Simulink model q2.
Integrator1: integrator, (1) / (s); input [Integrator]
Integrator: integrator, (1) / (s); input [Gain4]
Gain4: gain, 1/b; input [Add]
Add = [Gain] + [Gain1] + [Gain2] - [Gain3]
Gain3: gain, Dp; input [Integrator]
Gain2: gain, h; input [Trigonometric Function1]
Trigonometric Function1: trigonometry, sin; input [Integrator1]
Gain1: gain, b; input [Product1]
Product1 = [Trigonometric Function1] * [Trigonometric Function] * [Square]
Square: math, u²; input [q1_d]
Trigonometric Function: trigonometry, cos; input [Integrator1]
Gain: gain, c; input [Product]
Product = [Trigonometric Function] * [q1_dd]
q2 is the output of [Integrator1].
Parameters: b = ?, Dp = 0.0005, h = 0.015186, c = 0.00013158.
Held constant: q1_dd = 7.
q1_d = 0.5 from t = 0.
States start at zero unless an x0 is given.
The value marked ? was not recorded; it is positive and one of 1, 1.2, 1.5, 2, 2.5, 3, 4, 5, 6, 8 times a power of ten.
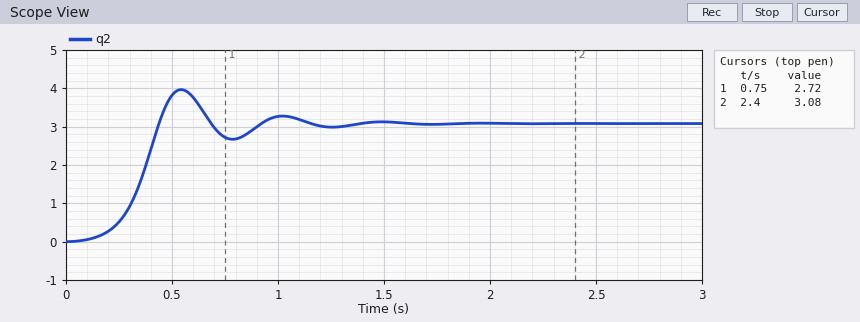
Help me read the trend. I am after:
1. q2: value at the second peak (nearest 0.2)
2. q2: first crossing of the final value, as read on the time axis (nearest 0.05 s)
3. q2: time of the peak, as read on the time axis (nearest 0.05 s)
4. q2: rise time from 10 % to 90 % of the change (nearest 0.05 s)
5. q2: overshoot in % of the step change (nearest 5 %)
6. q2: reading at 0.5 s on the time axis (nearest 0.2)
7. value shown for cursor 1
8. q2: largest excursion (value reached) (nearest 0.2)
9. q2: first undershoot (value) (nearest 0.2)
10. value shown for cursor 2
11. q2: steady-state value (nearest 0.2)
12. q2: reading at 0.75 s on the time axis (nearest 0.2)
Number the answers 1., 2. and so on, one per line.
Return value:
1. 3.2
2. 0.45 s
3. 0.55 s
4. 0.20 s
5. 30 %
6. 3.8
7. 2.72
8. 4.0
9. 2.6
10. 3.08
11. 3.0
12. 2.8
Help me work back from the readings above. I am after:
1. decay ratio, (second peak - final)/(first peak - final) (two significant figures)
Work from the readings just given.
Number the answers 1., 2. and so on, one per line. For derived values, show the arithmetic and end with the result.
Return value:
1. (3.2 - 3) / (4 - 3) = 0.20
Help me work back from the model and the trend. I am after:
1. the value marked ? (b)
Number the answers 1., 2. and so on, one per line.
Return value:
1. 8e-05
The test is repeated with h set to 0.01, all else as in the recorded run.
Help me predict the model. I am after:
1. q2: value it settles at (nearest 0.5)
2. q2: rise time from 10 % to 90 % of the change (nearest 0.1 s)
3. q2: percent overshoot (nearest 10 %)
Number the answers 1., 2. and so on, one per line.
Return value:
1. 3.0
2. 0.3 s
3. 20 %
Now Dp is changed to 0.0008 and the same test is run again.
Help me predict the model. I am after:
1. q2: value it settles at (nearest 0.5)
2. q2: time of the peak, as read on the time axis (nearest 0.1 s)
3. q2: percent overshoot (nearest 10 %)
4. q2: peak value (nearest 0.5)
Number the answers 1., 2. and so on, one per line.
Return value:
1. 3.0
2. 0.6 s
3. 20 %
4. 3.5
